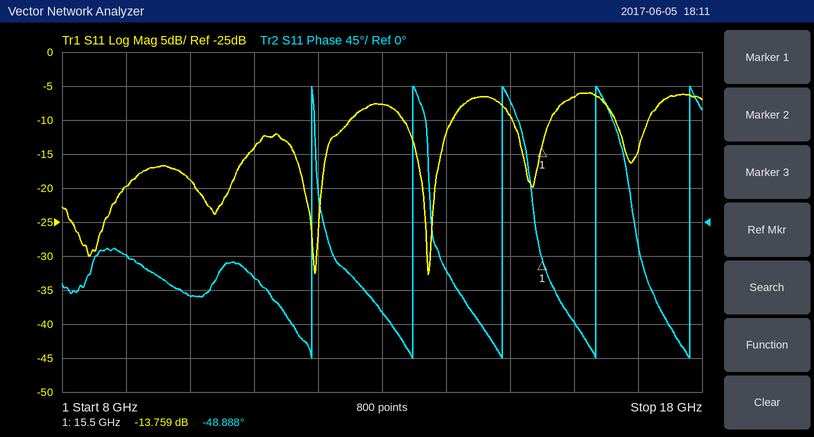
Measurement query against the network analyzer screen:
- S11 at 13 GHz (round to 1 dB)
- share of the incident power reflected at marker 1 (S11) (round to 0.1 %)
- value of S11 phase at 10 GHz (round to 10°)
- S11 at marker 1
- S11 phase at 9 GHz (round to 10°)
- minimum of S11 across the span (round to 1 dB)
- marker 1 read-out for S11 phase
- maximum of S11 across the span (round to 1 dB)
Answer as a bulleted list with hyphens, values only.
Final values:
- -8 dB
- 4.2 %
- -100°
- -13.759 dB
- -40°
- -33 dB
- -48.888°
- -6 dB
